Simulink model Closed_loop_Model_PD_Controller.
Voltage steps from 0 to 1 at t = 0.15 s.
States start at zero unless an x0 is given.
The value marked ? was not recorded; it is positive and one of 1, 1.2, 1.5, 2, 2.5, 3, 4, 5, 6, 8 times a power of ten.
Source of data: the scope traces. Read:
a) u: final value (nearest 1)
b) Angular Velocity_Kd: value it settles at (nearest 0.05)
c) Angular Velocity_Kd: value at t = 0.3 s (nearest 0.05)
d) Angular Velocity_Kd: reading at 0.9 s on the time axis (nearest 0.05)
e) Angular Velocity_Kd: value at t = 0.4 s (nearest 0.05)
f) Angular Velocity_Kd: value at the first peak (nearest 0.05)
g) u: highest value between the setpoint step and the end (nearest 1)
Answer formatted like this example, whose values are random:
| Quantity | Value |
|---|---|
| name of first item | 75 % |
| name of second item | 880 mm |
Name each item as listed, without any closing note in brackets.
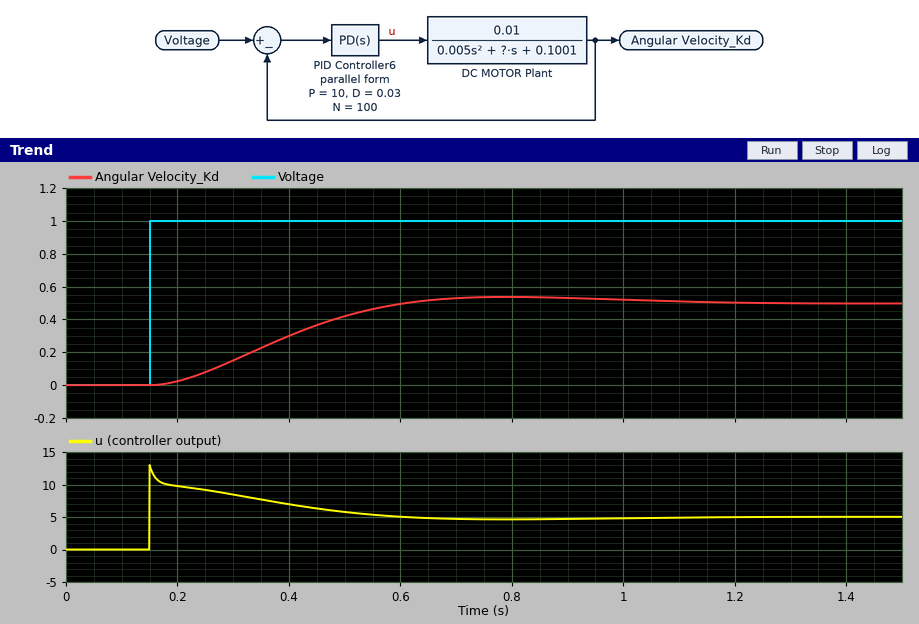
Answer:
| Quantity | Value |
|---|---|
| u: final value | 5 |
| Angular Velocity_Kd: value it settles at | 0.50 |
| Angular Velocity_Kd: value at t = 0.3 s | 0.15 |
| Angular Velocity_Kd: reading at 0.9 s on the time axis | 0.55 |
| Angular Velocity_Kd: value at t = 0.4 s | 0.30 |
| Angular Velocity_Kd: value at the first peak | 0.55 |
| u: highest value between the setpoint step and the end | 13 |
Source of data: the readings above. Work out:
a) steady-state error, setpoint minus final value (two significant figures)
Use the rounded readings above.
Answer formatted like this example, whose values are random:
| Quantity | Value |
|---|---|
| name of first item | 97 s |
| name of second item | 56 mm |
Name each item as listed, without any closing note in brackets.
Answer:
| Quantity | Value |
|---|---|
| steady-state error, setpoint minus final value | 0.50 |
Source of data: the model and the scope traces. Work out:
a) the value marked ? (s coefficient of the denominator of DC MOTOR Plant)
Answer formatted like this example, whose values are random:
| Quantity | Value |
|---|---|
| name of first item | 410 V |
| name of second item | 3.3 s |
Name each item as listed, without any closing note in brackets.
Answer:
| Quantity | Value |
|---|---|
| the value marked ? | 0.04 |
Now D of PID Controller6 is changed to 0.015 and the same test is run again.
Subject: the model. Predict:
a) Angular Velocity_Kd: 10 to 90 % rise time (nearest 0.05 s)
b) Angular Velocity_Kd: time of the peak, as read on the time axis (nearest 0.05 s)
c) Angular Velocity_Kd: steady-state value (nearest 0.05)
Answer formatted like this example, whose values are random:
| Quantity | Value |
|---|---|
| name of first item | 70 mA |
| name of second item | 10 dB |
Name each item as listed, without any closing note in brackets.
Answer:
| Quantity | Value |
|---|---|
| Angular Velocity_Kd: 10 to 90 % rise time | 0.30 s |
| Angular Velocity_Kd: time of the peak, as read on the time axis | 0.80 s |
| Angular Velocity_Kd: steady-state value | 0.50 |
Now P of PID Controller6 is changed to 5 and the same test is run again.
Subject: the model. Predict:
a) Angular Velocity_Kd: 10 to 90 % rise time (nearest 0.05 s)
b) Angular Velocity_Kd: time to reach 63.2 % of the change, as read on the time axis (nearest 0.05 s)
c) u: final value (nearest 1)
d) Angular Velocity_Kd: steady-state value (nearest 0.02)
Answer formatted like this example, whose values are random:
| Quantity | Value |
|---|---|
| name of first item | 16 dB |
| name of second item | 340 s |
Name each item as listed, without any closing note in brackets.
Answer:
| Quantity | Value |
|---|---|
| Angular Velocity_Kd: 10 to 90 % rise time | 0.40 s |
| Angular Velocity_Kd: time to reach 63.2 % of the change, as read on the time axis | 0.45 s |
| u: final value | 3 |
| Angular Velocity_Kd: steady-state value | 0.34 |
